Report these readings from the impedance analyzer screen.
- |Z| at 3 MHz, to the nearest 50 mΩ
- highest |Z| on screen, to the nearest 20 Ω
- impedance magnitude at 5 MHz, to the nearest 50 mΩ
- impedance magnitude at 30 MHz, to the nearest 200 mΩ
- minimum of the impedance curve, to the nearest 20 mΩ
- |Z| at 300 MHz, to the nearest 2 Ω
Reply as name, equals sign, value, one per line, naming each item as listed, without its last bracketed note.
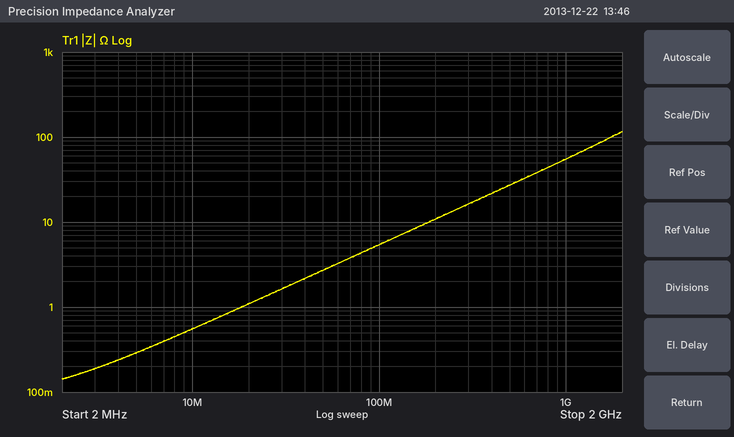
|Z| at 3 MHz, to the nearest 50 mΩ = 200 mΩ
highest |Z| on screen, to the nearest 20 Ω = 120 Ω
impedance magnitude at 5 MHz, to the nearest 50 mΩ = 300 mΩ
impedance magnitude at 30 MHz, to the nearest 200 mΩ = 1.6 Ω
minimum of the impedance curve, to the nearest 20 mΩ = 140 mΩ
|Z| at 300 MHz, to the nearest 2 Ω = 16 Ω
